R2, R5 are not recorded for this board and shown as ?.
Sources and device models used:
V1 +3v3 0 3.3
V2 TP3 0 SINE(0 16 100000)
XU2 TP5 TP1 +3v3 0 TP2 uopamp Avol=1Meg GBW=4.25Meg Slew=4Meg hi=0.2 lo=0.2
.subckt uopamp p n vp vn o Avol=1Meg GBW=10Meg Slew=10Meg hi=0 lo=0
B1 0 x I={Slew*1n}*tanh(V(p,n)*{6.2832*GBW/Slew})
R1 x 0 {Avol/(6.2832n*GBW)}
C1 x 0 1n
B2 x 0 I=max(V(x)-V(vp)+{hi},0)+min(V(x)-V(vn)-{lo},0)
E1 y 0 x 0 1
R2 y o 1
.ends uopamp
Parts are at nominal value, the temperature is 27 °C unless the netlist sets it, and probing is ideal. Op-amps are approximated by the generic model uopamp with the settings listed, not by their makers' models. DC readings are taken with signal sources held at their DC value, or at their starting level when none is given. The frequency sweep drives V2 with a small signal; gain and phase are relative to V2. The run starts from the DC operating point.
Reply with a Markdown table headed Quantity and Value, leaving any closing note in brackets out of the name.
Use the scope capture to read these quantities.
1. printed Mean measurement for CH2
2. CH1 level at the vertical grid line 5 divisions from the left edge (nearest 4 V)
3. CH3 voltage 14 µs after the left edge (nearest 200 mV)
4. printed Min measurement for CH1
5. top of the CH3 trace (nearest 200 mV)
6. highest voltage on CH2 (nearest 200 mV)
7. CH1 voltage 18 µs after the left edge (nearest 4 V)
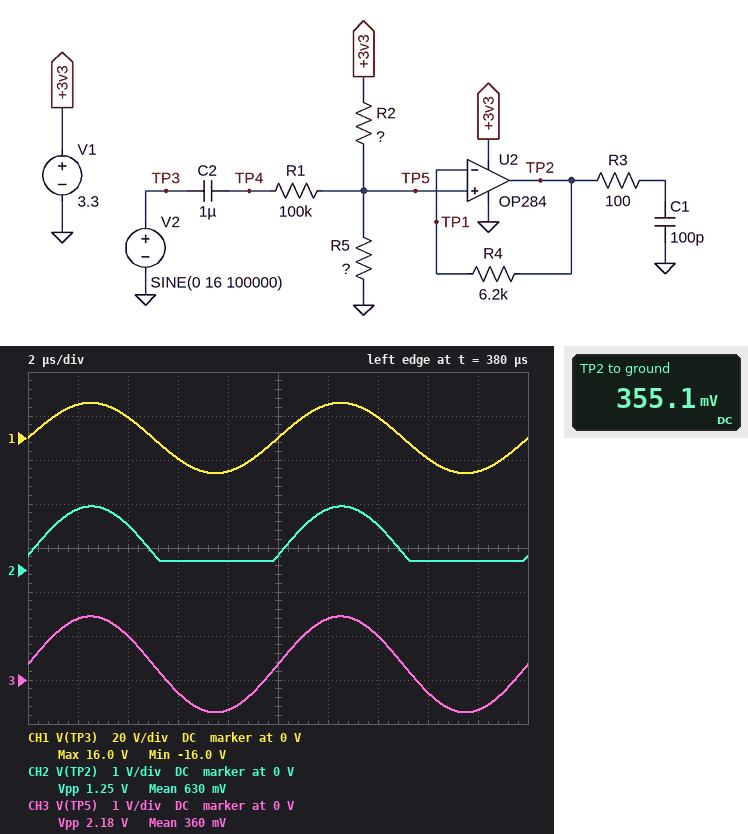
| Quantity | Value |
|---|---|
| printed Mean measurement for CH2 | 630 mV |
| CH1 level at the vertical grid line 5 divisions from the left edge | 0 V |
| CH3 voltage 14 µs after the left edge | 1.0 V |
| printed Min measurement for CH1 | -16.0 V |
| top of the CH3 trace | 1.4 V |
| highest voltage on CH2 | 1.4 V |
| CH1 voltage 18 µs after the left edge | -16 V |
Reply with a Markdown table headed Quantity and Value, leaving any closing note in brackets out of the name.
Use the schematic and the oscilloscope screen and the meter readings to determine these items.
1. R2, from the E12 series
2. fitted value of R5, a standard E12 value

| Quantity | Value |
|---|---|
| R2, from the E12 series | 68 kΩ |
| fitted value of R5, a standard E12 value | 8.2 kΩ |
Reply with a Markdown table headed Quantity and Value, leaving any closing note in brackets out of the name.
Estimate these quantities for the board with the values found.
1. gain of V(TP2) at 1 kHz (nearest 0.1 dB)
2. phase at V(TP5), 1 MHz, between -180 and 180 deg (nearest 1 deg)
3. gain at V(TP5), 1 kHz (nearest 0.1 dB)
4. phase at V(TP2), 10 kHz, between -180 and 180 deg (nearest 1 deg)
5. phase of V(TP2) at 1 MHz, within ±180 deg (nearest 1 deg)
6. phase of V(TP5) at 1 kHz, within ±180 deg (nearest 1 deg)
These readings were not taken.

| Quantity | Value |
|---|---|
| gain of V(TP2) at 1 kHz | -23.3 dB |
| phase at V(TP5), 1 MHz, between -180 and 180 deg | 0 deg |
| gain at V(TP5), 1 kHz | -23.3 dB |
| phase at V(TP2), 10 kHz, between -180 and 180 deg | 0 deg |
| phase of V(TP2) at 1 MHz, within ±180 deg | -13 deg |
| phase of V(TP5) at 1 kHz, within ±180 deg | 0 deg |
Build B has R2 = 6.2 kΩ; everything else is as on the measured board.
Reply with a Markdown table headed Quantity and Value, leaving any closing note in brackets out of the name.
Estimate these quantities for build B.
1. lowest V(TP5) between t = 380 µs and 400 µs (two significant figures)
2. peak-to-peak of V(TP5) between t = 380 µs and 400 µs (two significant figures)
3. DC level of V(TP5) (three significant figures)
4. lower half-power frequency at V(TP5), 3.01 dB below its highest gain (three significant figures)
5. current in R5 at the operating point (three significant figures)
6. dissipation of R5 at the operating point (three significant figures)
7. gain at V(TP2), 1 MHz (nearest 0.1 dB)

| Quantity | Value |
|---|---|
| lowest V(TP5) between t = 380 µs and 400 µs | 1.3 V |
| peak-to-peak of V(TP5) between t = 380 µs and 400 µs | 1.1 V |
| DC level of V(TP5) | 1.88 V |
| lower half-power frequency at V(TP5), 3.01 dB below its highest gain | 1.54 Hz |
| current in R5 at the operating point | 229 µA |
| dissipation of R5 at the operating point | 431 µW |
| gain at V(TP2), 1 MHz | -29.6 dB |
